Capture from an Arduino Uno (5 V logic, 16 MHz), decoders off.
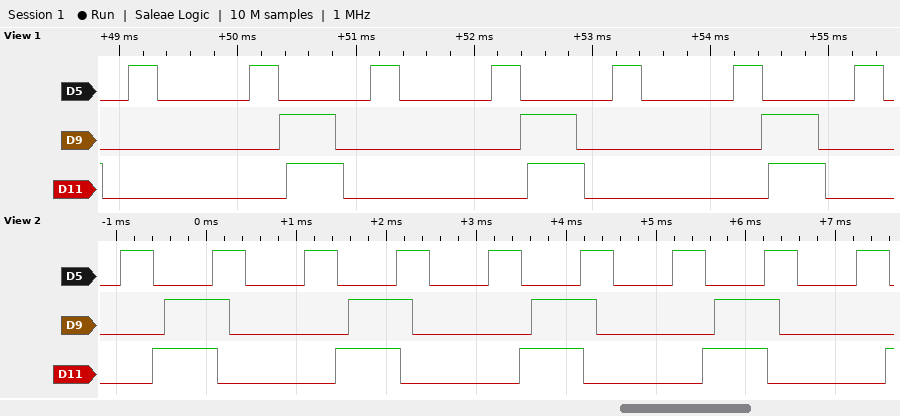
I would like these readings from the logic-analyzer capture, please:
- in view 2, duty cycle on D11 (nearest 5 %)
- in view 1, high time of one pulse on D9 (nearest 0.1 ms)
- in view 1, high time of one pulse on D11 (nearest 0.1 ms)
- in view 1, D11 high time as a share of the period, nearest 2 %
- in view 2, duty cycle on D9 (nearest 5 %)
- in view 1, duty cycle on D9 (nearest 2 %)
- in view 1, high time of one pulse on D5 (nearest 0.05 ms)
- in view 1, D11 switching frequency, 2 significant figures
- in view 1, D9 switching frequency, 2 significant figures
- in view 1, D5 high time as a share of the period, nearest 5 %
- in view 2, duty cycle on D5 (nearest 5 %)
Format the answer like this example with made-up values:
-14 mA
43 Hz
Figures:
35 %
0.5 ms
0.5 ms
24 %
35 %
24 %
0.25 ms
490 Hz
490 Hz
25 %
35 %
